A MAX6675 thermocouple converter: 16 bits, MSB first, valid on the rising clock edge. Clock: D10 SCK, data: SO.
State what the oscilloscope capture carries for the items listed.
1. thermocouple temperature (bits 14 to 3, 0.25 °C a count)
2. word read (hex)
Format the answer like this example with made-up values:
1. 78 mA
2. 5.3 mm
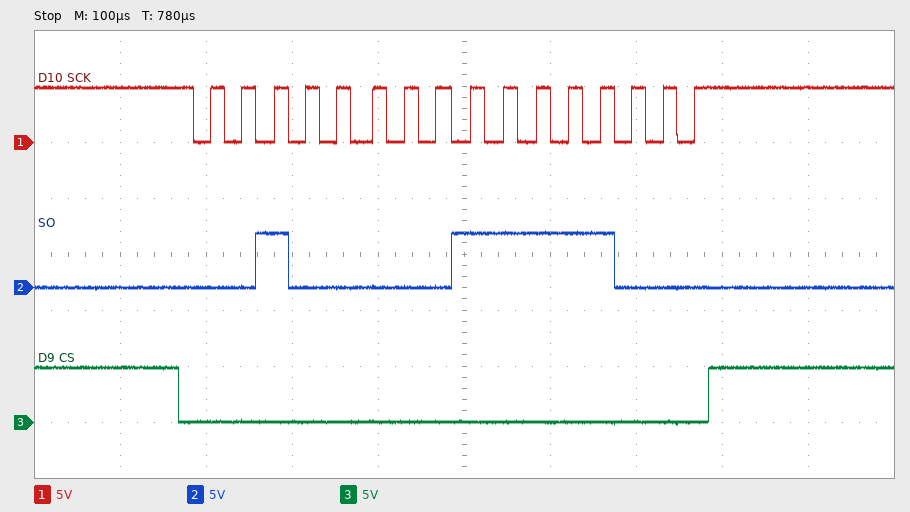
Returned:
1. 263.75 °C
2. 0x20F8
